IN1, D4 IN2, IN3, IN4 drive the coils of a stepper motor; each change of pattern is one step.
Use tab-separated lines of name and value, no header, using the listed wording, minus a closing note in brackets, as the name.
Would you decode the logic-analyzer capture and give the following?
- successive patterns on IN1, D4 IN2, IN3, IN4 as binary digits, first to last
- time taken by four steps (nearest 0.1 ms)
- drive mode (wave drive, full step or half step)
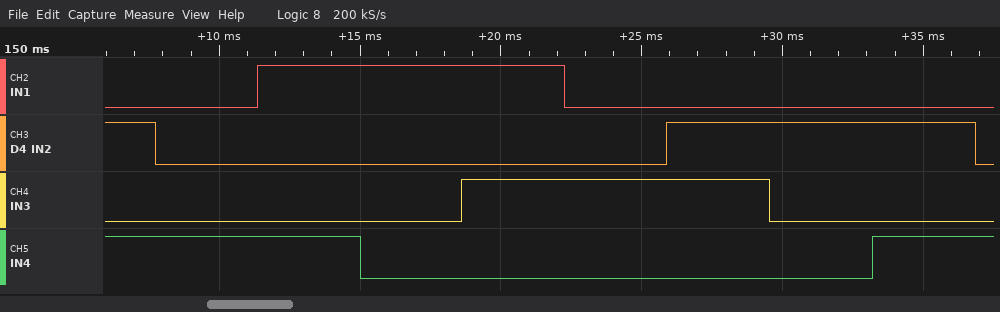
successive patterns on IN1, D4 IN2, IN3, IN4 as binary digits, first to last	0101 0001 1001 1000 1010 0010 0110 0100 0101 0001
time taken by four steps	14.5 ms
drive mode	half step
